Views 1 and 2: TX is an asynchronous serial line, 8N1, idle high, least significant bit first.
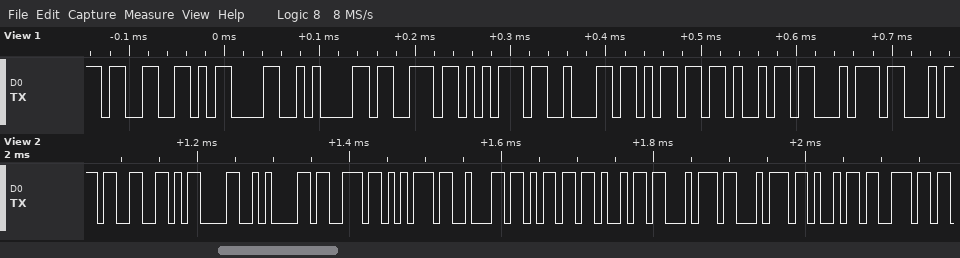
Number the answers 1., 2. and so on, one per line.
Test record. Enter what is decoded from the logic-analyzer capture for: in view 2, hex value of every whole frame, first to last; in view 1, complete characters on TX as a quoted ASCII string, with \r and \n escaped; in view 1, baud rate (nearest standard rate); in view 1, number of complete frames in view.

1. 0x33 0x0D 0x0A 0x73 0x75 0x62 0x6D 0x69 0x74 0x74 0x69 0x6E
2. "3\r\nsubmit"
3. 115200 baud
4. 9
